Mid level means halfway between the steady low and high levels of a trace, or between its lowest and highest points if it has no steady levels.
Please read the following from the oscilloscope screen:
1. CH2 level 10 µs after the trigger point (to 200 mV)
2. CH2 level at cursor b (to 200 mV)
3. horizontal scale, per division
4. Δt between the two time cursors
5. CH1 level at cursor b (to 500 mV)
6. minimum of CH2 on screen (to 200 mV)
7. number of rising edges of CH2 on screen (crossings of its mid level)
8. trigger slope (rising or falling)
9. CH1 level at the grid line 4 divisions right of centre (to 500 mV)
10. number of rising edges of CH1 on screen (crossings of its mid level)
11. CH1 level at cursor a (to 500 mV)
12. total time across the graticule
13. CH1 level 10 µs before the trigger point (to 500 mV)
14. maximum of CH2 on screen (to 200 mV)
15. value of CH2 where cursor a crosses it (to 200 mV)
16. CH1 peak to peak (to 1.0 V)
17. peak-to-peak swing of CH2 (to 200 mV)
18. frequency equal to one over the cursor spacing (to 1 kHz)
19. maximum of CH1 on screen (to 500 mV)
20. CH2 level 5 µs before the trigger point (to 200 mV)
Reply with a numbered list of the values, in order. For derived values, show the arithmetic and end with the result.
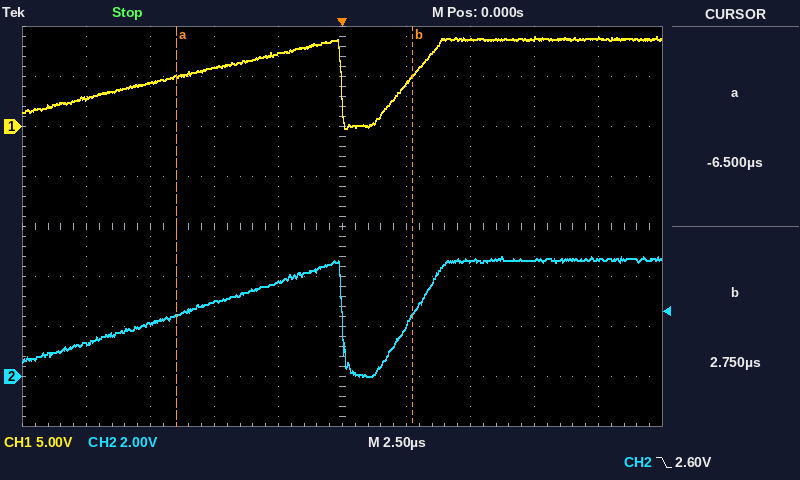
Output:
1. 4.6 V
2. 2.4 V
3. 2.5 µs
4. 2.75 µs − (-6.5 µs) = 9.25 µs
5. 5.0 V
6. 0.0 V
7. 2
8. falling
9. 9.0 V
10. 2
11. 5.0 V
12. 25 µs
13. 3.0 V
14. 4.8 V
15. 2.4 V
16. 9.0 V
17. 4.8 V − (0.0 V) = 4.8 V
18. 1 / 9.25 µs ≈ 108 kHz
19. 9.0 V
20. 3.0 V
